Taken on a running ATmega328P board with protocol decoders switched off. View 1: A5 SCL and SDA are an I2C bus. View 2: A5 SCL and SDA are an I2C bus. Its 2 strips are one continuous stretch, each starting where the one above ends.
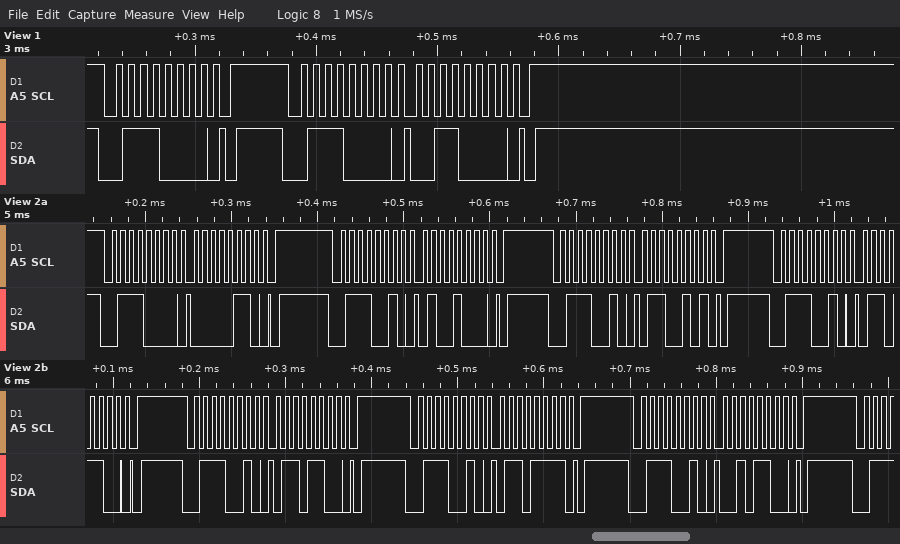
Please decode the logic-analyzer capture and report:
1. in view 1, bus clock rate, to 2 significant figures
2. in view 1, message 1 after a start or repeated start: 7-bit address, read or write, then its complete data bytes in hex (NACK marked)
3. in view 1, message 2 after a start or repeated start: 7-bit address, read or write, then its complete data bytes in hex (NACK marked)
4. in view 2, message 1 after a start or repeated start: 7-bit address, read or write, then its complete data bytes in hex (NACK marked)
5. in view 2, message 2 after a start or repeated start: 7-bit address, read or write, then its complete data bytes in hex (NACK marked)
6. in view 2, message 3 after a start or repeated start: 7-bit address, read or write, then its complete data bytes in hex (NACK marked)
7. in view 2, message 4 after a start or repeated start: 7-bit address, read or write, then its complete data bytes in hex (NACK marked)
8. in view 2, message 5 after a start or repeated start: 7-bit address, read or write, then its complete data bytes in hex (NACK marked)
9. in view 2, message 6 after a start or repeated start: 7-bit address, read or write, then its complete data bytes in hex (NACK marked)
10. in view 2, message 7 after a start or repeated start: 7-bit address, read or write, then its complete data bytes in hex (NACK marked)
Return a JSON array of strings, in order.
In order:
["100 kHz", "0x38 write", "0x38 write: 30", "0x38 write: 06", "0x39 write: 48", "0x39 write: 65", "0x39 write: 6C", "0x39 write: 6C", "0x39 write: 6F", "0x39 write: 2C"]
